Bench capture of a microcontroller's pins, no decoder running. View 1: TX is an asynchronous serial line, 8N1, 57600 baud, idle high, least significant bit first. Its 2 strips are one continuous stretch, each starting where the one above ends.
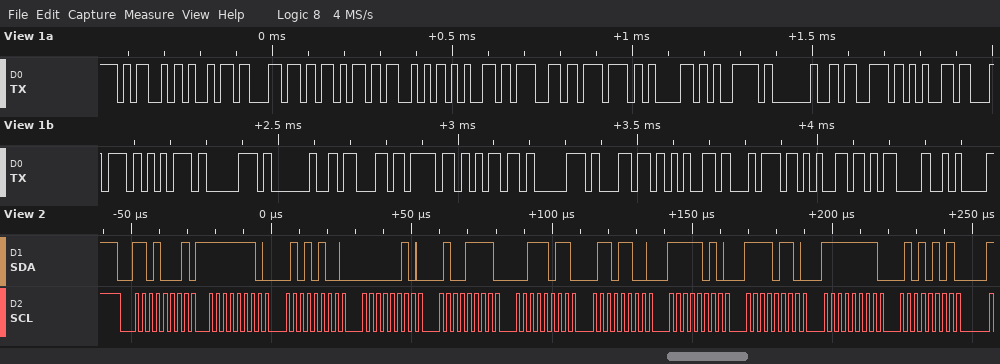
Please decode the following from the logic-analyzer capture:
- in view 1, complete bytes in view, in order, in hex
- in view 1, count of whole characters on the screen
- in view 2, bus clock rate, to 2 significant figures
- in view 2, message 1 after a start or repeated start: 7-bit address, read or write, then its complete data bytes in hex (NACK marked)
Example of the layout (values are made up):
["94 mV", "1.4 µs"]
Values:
["4D 69 6C 6B 53 65 67 77 61 79 20 73 65 74 75 70 20 63 6F 6D 70 6C 65 74 65 0D 0A", "27", "400 kHz", "0x68 read: FE 54 02 4F 3B 6C FA F6 FF 55"]
